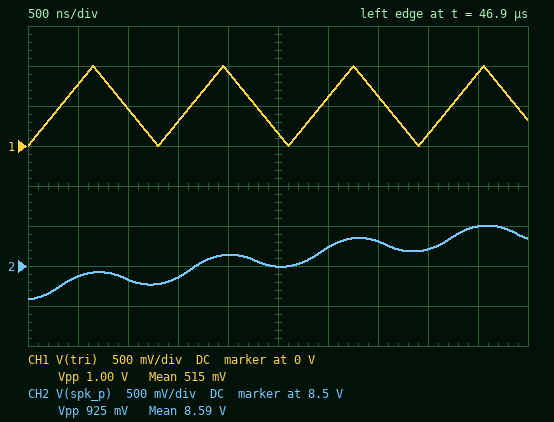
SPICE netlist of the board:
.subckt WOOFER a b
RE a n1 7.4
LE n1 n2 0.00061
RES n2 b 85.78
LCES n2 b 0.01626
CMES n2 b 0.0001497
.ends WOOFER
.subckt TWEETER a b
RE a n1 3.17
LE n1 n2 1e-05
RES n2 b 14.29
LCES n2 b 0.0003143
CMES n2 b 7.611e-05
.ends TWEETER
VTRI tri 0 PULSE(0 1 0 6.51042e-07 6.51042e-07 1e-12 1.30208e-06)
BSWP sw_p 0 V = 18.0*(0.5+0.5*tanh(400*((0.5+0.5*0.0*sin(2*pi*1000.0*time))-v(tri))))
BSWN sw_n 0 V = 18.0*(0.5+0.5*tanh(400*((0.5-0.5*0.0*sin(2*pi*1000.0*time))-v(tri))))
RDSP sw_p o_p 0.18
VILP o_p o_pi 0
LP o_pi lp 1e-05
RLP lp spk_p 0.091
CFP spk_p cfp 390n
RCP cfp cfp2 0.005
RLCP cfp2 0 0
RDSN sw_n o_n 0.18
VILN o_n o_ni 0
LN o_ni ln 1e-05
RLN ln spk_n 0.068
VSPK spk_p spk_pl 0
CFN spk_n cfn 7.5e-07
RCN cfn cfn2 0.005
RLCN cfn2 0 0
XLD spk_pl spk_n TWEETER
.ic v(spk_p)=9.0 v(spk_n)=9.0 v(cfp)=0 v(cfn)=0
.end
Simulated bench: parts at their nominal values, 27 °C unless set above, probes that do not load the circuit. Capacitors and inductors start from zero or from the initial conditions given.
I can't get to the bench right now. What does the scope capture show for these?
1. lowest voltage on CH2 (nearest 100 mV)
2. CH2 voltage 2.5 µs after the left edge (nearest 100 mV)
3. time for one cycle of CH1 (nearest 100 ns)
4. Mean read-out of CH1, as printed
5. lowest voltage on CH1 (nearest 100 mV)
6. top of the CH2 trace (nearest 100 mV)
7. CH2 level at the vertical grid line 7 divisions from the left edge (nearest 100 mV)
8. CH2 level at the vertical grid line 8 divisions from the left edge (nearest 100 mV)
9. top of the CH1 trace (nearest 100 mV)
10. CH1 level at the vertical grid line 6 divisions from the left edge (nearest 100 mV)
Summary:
8.1 V
8.5 V
1.3 µs
515 mV
0 V
9.0 V
8.8 V
8.7 V
1.0 V
600 mV
